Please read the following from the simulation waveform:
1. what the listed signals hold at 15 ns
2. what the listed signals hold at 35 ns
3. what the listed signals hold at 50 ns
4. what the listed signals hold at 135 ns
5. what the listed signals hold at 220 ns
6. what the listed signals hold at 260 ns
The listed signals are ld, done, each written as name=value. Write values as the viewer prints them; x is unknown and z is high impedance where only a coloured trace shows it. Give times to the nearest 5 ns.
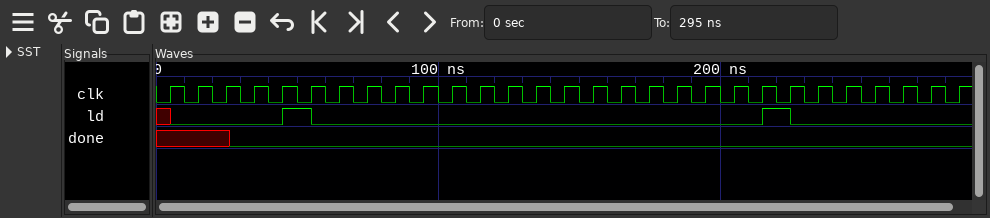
ld=0, done=x
ld=0, done=0
ld=1, done=0
ld=0, done=0
ld=1, done=0
ld=0, done=0
